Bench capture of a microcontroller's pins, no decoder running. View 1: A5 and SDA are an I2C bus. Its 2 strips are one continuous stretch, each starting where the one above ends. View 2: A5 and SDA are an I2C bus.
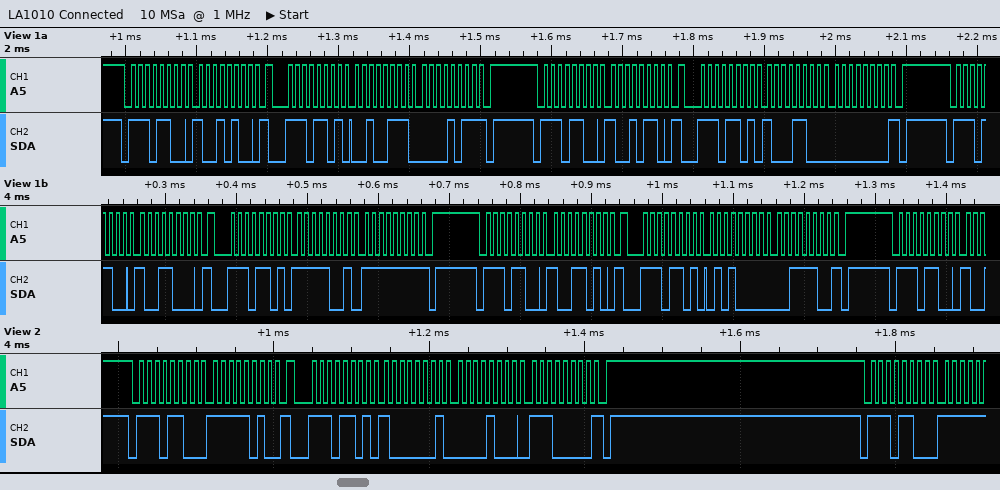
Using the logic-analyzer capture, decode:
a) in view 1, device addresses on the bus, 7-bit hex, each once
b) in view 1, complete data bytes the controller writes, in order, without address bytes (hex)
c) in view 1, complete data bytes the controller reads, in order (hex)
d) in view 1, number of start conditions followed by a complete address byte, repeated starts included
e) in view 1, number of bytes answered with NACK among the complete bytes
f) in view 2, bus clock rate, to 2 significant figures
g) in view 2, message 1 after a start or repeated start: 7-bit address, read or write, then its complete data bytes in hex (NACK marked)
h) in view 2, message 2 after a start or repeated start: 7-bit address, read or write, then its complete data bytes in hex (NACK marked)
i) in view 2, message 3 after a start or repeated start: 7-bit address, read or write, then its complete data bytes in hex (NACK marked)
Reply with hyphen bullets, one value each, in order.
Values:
- 0x76
- 94 96 98 9A
- 27 0B 8C 00 F9 FF 50 3C
- 9
- 4
- 100 kHz
- 0x76 write: FA
- 0x76 read: 81 08 E0 NACK
- 0x76 write
